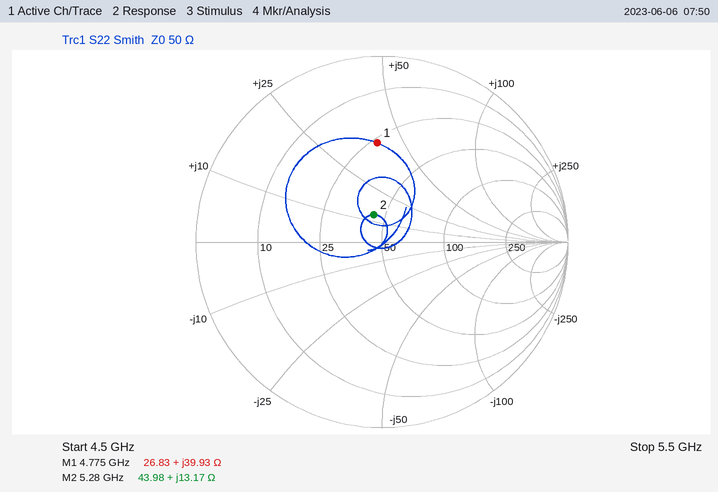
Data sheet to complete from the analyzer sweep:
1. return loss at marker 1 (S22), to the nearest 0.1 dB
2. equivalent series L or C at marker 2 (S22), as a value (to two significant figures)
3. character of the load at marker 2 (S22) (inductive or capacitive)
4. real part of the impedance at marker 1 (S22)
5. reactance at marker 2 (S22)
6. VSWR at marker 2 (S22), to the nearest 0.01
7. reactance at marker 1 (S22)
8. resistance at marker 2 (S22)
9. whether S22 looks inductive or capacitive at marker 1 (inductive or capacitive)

5.5 dB
400 pH
inductive
26.83 Ω
+13.17 Ω
1.36
+39.93 Ω
43.98 Ω
inductive
